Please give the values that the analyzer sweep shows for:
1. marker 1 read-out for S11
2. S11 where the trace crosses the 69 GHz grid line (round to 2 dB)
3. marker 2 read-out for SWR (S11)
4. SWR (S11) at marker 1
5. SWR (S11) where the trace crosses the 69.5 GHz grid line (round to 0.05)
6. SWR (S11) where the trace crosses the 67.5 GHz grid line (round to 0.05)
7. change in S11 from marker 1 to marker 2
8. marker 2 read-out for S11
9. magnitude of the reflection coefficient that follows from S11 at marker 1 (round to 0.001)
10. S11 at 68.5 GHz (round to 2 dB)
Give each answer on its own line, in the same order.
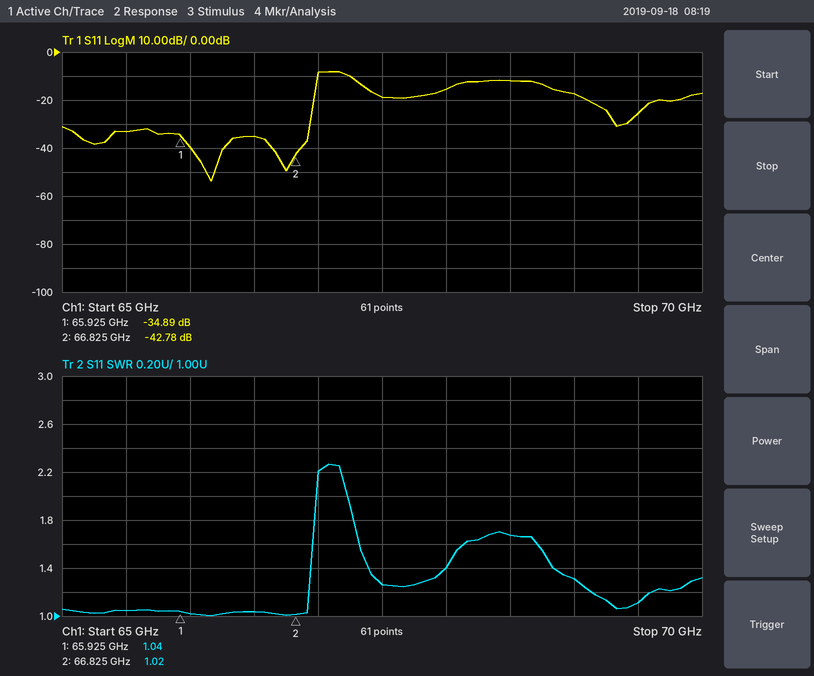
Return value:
-34.89 dB
-18 dB
1.02
1.04
1.10
1.25
-7.89 dB
-42.78 dB
0.018
-12 dB
